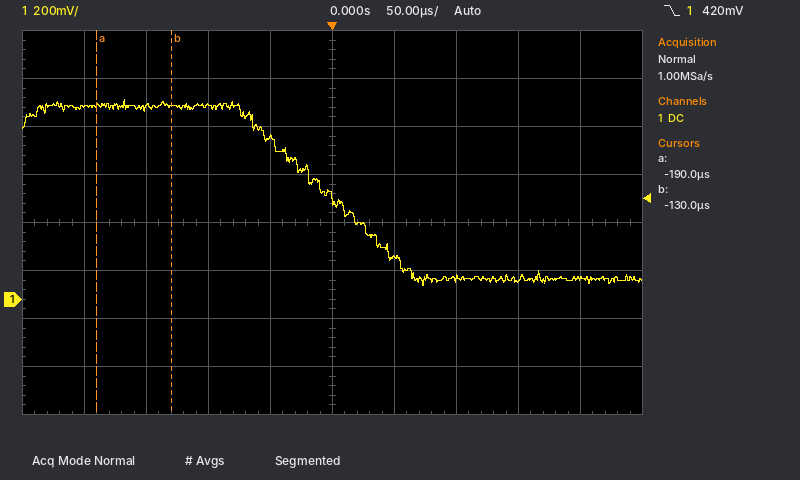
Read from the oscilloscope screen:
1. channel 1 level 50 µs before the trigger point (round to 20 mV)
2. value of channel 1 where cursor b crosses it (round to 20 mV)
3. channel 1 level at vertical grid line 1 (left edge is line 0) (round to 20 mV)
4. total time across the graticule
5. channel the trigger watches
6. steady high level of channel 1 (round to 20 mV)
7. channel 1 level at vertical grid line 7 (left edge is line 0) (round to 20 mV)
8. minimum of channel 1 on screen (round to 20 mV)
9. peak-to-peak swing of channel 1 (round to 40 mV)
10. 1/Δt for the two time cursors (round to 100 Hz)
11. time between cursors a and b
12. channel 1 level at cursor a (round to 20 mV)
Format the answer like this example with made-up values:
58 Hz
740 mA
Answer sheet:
680 mV
800 mV
800 mV
500 µs
channel 1
800 mV
80 mV
60 mV
760 mV
16.7 kHz
60 µs
800 mV
